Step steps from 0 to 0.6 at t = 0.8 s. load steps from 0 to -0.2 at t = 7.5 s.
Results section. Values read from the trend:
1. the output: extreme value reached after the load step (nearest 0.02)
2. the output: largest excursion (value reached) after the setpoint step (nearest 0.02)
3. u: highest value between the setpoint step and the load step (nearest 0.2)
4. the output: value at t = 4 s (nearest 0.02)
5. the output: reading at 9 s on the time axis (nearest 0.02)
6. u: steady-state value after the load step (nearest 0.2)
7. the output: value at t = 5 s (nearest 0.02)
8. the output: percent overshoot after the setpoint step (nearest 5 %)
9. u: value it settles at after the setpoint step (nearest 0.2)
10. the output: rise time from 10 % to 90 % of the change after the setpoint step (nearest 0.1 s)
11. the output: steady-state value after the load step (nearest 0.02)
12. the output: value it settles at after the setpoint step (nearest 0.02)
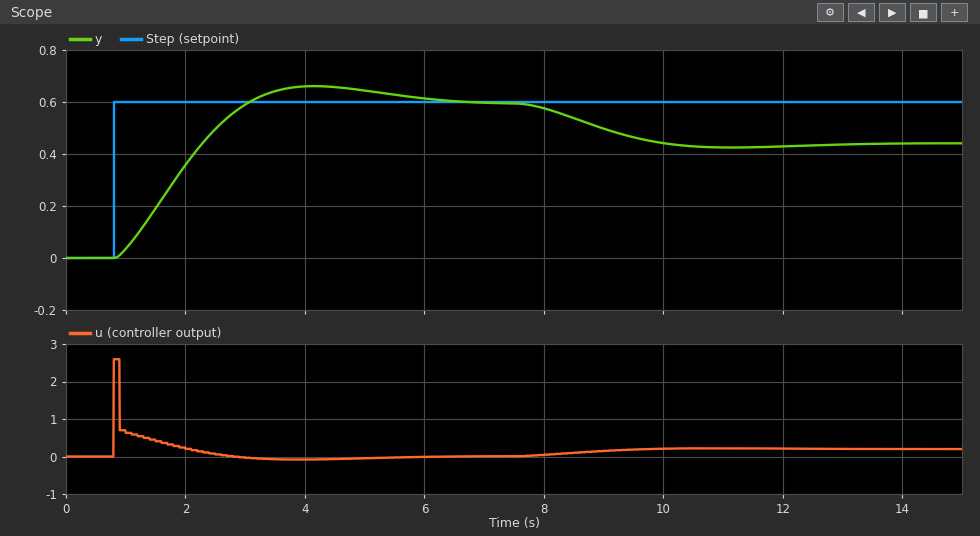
0.42
0.66
2.6
0.66
0.50
0.2
0.64
10 %
0.0
1.6 s
0.44
0.60
